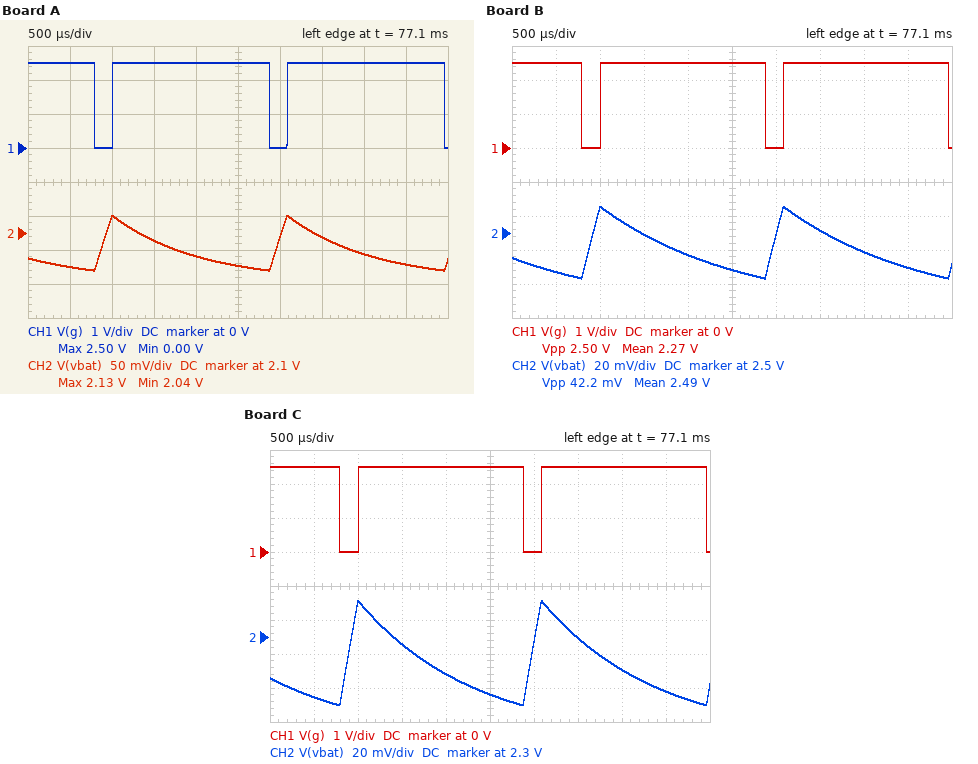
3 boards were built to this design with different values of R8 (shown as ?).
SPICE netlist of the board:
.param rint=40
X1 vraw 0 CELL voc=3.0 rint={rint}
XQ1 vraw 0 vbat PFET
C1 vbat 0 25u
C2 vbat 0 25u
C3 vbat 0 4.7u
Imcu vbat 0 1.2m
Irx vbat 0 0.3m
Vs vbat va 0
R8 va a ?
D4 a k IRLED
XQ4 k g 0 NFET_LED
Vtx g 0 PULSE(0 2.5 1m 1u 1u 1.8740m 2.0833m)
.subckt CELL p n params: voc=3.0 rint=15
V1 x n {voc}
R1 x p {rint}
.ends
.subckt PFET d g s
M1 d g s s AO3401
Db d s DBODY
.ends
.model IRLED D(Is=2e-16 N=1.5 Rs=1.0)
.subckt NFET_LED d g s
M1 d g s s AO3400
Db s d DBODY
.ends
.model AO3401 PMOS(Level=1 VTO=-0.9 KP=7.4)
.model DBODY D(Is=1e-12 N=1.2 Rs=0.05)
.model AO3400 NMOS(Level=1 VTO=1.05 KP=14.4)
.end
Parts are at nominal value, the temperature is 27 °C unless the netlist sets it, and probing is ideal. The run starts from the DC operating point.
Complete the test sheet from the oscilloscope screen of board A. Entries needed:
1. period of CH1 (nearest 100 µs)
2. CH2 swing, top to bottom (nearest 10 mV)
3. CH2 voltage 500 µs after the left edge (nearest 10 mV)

2.1 ms
80 mV
2.05 V
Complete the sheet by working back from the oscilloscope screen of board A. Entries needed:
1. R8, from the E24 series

33 Ω
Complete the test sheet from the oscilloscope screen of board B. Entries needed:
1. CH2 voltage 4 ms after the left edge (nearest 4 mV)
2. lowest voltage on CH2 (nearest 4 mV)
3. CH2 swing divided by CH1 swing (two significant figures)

2.488 V
2.472 V
0.017
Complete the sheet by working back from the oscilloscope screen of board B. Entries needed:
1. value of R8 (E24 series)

100 Ω
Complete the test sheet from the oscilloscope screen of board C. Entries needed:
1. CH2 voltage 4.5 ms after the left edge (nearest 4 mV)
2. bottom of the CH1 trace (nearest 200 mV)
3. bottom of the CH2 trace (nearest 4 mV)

2.268 V
0 V
2.260 V
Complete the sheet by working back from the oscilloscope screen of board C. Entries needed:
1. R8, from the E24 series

56 Ω
